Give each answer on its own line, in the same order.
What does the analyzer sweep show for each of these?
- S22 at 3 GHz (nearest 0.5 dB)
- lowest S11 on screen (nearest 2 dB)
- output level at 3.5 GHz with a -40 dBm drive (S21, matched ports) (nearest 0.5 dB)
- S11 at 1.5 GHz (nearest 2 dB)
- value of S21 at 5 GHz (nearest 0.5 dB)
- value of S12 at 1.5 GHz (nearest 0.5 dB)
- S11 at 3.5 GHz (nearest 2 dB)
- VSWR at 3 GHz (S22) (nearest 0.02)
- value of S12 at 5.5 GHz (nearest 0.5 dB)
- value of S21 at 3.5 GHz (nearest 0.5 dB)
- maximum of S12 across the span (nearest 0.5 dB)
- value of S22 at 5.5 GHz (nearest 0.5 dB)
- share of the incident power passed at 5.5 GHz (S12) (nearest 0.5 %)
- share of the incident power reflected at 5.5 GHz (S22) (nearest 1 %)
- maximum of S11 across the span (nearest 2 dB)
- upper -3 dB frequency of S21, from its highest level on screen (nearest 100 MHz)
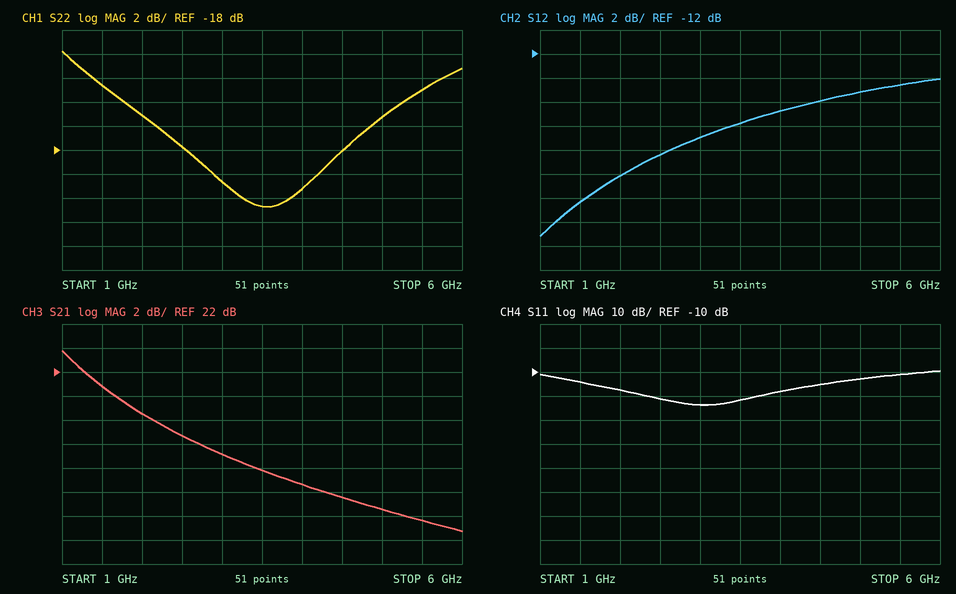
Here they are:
-20.5 dB
-24 dB
-26.0 dBm
-14 dB
10.5 dB
-24.5 dB
-22 dB
1.20
-14.5 dB
14.0 dB
-14.0 dB
-13.0 dB
3.5 %
5 %
-10 dB
1.5 GHz
